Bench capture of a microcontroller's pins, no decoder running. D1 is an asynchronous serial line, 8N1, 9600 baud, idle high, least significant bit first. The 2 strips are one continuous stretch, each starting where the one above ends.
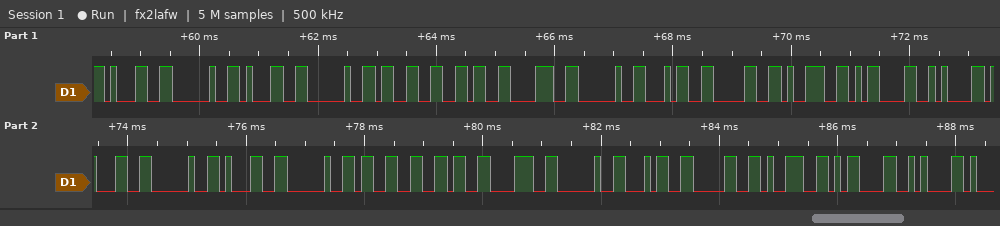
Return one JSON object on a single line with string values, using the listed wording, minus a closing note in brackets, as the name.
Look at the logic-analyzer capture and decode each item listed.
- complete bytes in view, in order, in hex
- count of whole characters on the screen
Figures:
{"complete bytes in view, in order, in hex": "31 20 31 20 33 36 38 20 34 30 39 0D 0A 31 20 31 20 33 36 38 20 34 30 39 0D 0A", "count of whole characters on the screen": "26"}
